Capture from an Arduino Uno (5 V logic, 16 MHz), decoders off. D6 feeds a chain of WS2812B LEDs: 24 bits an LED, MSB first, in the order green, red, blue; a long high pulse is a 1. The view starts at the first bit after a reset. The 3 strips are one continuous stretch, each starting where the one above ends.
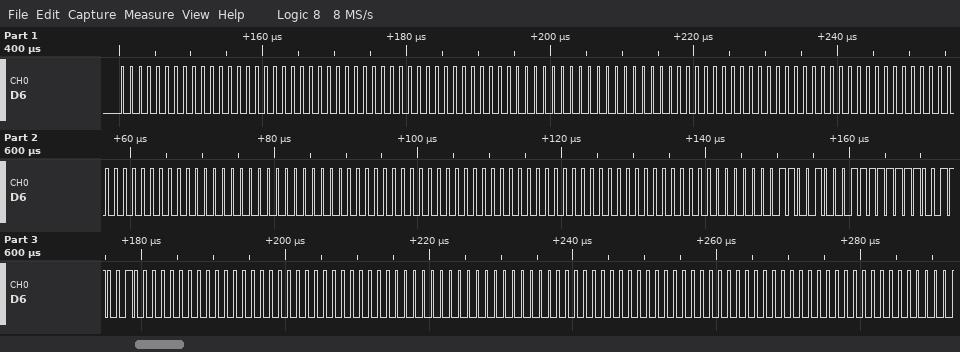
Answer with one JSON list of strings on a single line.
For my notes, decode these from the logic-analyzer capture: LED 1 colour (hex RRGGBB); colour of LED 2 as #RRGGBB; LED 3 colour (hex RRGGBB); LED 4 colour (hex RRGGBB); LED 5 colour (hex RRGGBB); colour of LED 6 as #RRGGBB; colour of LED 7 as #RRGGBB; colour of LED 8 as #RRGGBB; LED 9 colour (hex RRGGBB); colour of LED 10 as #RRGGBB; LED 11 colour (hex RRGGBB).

["#000000", "#000000", "#000000", "#000000", "#000000", "#000000", "#000000", "#FFC832", "#000000", "#000000", "#000000"]
